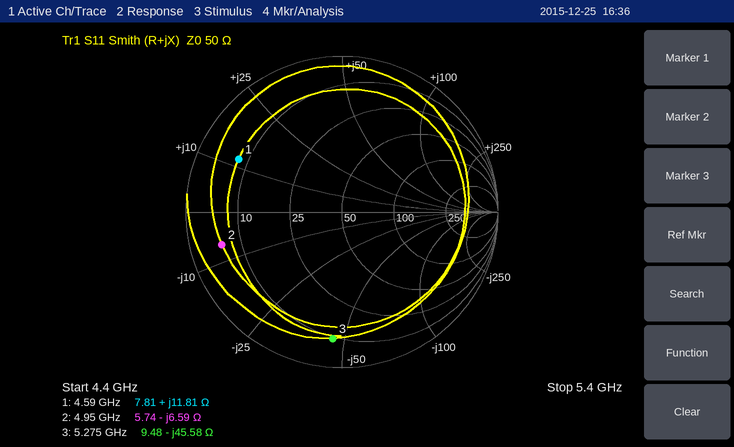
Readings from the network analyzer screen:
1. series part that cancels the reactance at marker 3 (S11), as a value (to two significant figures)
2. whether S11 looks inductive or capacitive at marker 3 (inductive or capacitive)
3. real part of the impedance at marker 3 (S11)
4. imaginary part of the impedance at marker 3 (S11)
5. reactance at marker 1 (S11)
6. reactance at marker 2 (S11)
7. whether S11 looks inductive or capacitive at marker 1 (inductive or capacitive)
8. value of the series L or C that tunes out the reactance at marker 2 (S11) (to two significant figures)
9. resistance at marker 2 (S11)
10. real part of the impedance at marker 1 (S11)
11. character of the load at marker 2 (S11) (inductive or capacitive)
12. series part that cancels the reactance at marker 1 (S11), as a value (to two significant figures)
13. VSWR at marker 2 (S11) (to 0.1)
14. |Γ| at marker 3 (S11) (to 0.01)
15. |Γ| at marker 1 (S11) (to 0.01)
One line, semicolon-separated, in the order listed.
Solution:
1.4 nH; capacitive; 9.48 Ω; -45.58 Ω; +11.81 Ω; -6.59 Ω; inductive; 210 pH; 5.74 Ω; 7.81 Ω; capacitive; 2.9 pF; 8.9; 0.81; 0.74
